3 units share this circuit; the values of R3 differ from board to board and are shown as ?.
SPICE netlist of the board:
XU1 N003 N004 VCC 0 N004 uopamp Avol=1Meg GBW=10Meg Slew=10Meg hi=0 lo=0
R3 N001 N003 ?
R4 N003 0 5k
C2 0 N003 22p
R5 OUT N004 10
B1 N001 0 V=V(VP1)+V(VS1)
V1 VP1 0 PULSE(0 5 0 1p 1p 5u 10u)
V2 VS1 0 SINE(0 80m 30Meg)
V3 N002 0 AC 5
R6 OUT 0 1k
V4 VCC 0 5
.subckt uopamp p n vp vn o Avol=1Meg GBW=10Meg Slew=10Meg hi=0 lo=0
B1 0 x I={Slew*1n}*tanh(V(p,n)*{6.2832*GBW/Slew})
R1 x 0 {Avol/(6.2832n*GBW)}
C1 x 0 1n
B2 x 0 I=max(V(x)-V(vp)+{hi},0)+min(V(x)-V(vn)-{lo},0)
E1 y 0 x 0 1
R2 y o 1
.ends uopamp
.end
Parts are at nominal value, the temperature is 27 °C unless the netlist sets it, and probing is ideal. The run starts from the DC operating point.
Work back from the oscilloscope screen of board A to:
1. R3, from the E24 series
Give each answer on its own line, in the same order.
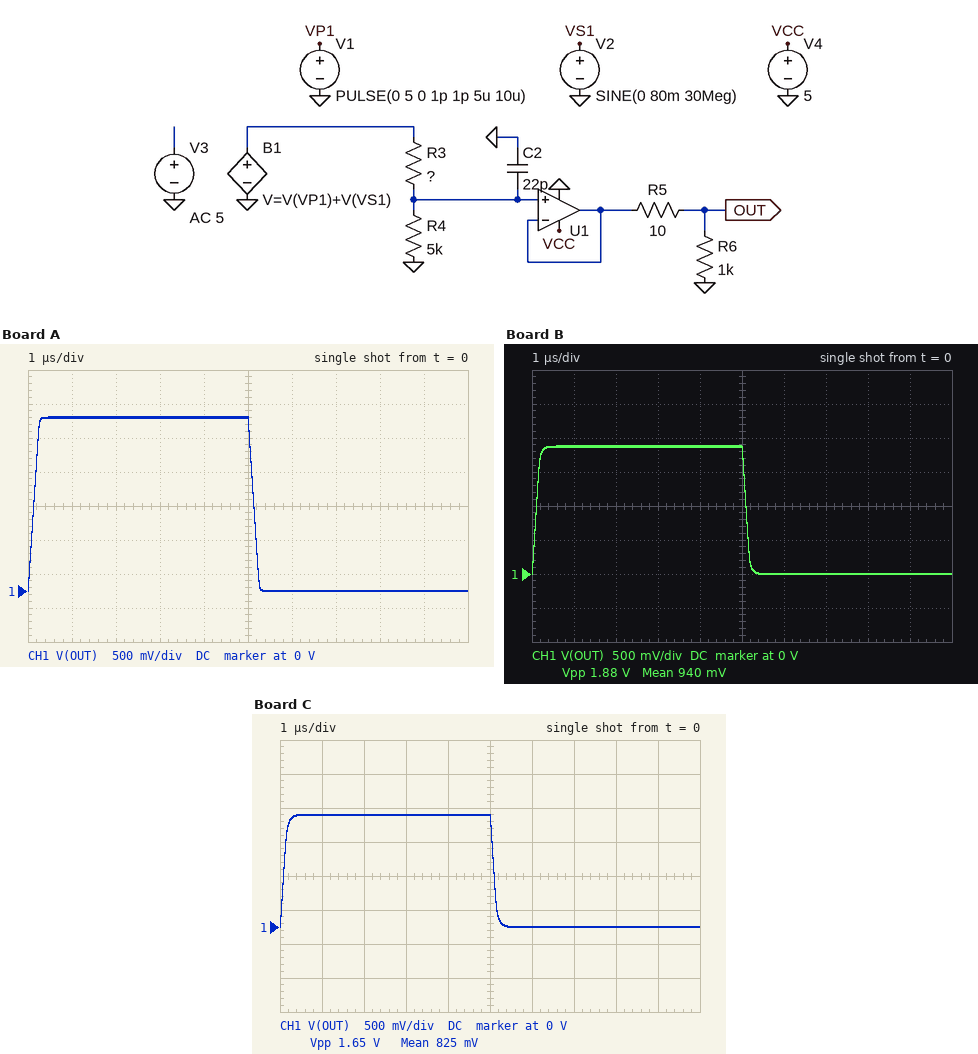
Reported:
4.7 kΩ
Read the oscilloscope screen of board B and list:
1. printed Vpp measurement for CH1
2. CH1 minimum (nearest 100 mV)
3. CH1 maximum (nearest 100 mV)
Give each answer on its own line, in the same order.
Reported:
1.88 V
0 V
1.9 V
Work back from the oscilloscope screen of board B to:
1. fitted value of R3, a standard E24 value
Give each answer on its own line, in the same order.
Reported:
8.2 kΩ
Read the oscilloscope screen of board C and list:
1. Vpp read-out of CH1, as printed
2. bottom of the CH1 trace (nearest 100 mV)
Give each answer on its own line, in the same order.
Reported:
1.65 V
0 V
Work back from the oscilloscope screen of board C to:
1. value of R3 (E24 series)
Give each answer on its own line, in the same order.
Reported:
10 kΩ
